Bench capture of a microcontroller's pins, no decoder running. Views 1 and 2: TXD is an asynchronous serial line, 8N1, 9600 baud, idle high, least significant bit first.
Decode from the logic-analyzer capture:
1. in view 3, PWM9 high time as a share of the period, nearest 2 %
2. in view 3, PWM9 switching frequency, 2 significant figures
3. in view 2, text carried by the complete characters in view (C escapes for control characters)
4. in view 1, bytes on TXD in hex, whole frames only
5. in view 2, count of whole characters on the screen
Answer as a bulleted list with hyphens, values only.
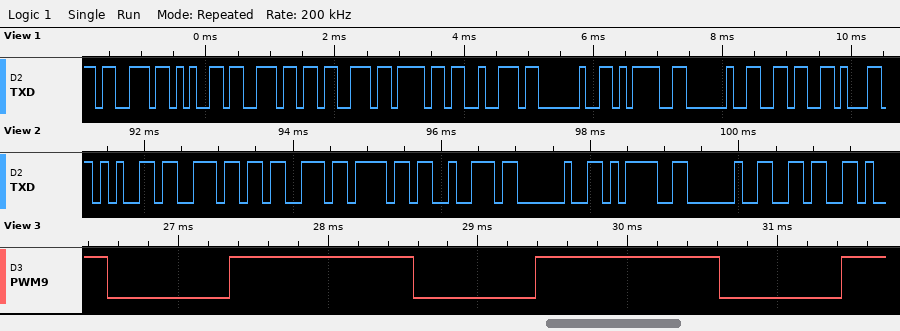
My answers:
- 60 %
- 490 Hz
- "ensor = 6"
- 0x73 0x65 0x6E 0x73 0x6F 0x72 0x20 0x3D 0x20 0x36
- 9
